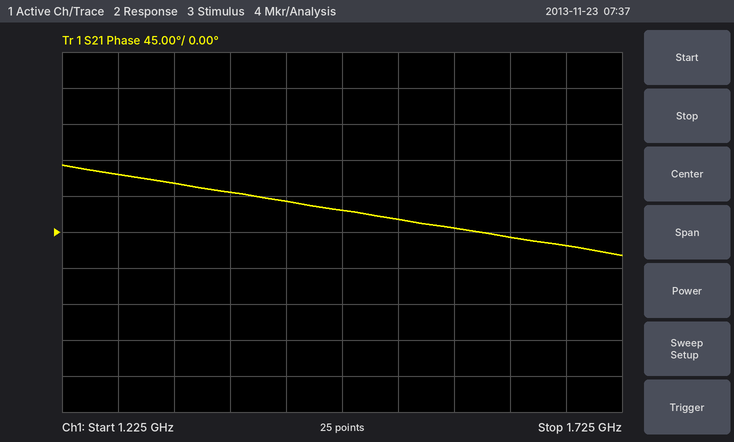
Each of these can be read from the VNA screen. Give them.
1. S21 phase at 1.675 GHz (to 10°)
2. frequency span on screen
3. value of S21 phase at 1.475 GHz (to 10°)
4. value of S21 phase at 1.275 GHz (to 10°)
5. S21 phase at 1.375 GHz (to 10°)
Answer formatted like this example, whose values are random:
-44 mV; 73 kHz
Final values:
-20°; 500 MHz; 30°; 70°; 50°
